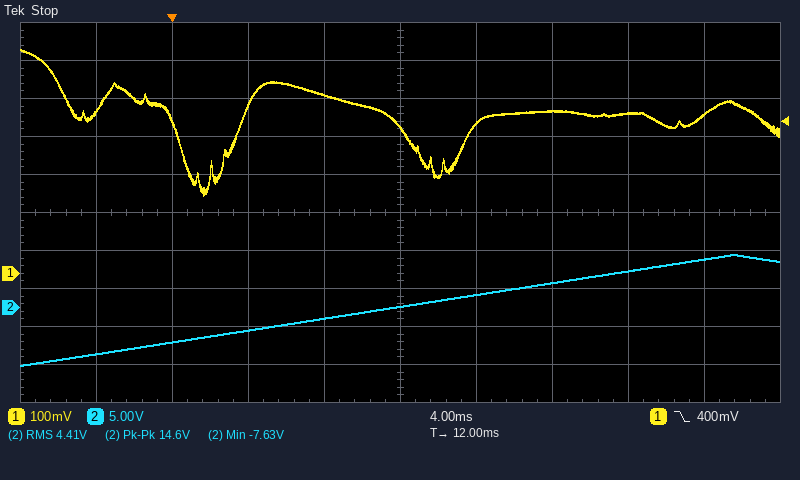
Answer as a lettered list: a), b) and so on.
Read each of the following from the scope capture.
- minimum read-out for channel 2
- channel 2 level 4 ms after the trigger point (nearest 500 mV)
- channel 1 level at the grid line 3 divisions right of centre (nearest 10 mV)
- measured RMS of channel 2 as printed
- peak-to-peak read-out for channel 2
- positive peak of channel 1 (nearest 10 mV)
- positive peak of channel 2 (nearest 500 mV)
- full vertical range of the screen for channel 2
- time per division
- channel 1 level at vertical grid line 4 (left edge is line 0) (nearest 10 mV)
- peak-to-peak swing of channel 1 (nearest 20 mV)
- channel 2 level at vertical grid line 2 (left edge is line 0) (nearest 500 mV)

a) -7.63 V
b) -3.0 V
c) 420 mV
d) 4.41 V
e) 14.6 V
f) 590 mV
g) 7.0 V
h) 50 V
i) 4 ms
j) 470 mV
k) 380 mV
l) -4.5 V
